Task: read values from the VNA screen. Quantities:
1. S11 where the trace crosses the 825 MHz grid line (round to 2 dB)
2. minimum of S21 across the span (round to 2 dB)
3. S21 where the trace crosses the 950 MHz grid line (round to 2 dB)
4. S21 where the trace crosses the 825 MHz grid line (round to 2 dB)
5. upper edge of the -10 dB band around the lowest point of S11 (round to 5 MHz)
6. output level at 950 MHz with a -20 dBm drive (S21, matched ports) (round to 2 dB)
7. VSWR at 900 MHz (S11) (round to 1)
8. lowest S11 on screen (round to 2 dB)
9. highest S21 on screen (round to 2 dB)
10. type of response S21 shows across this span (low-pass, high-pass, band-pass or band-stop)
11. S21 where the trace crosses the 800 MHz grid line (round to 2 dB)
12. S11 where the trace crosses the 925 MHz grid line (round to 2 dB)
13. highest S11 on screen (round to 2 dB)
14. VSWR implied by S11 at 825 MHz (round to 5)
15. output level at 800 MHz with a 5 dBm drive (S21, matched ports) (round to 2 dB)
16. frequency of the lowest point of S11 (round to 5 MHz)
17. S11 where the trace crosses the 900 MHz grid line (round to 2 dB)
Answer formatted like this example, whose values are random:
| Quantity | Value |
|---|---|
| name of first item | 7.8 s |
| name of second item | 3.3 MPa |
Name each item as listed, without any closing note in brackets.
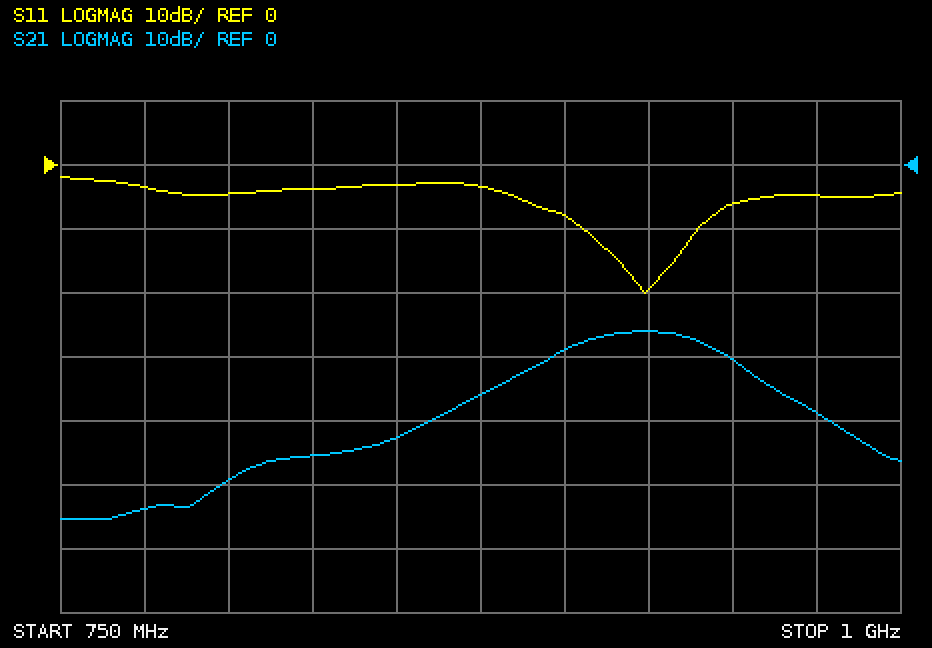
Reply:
| Quantity | Value |
|---|---|
| S11 where the trace crosses the 825 MHz grid line | -4 dB |
| minimum of S21 across the span | -56 dB |
| S21 where the trace crosses the 950 MHz grid line | -30 dB |
| S21 where the trace crosses the 825 MHz grid line | -46 dB |
| upper edge of the -10 dB band around the lowest point of S11 | 940 MHz |
| output level at 950 MHz with a -20 dBm drive (S21, matched ports) | -50 dBm |
| VSWR at 900 MHz (S11) | 2 |
| lowest S11 on screen | -20 dB |
| highest S21 on screen | -26 dB |
| type of response S21 shows across this span | band-pass |
| S21 where the trace crosses the 800 MHz grid line | -50 dB |
| S11 where the trace crosses the 925 MHz grid line | -20 dB |
| highest S11 on screen | -2 dB |
| VSWR implied by S11 at 825 MHz | 5 |
| output level at 800 MHz with a 5 dBm drive (S21, matched ports) | -44 dBm |
| frequency of the lowest point of S11 | 925 MHz |
| S11 where the trace crosses the 900 MHz grid line | -8 dB |
